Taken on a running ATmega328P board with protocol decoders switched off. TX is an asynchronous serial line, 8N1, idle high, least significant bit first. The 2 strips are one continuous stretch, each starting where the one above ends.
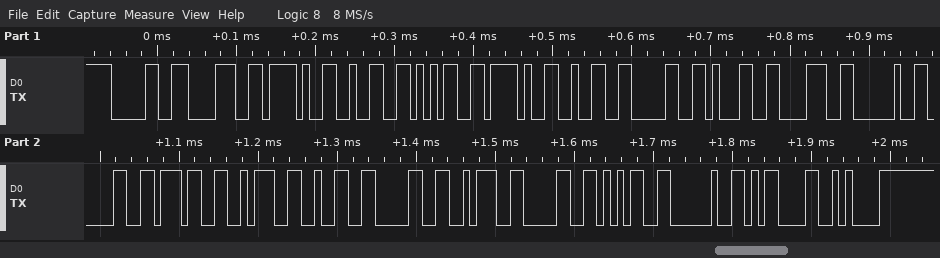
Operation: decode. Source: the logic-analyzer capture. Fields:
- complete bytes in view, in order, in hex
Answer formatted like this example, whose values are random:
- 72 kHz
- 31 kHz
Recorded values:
- 0x30 0x38 0x2F 0x32 0x35 0x2F 0x32 0x30 0x31 0x38 0x20 0x30 0x37 0x3A 0x32 0x30 0x3A 0x30 0x35 0x20 0x0D 0x0A
